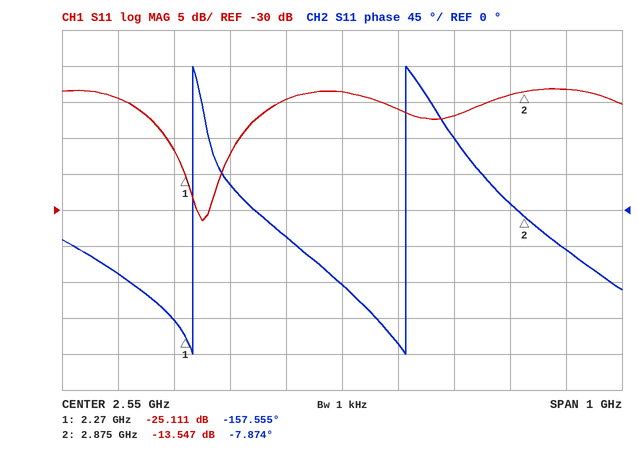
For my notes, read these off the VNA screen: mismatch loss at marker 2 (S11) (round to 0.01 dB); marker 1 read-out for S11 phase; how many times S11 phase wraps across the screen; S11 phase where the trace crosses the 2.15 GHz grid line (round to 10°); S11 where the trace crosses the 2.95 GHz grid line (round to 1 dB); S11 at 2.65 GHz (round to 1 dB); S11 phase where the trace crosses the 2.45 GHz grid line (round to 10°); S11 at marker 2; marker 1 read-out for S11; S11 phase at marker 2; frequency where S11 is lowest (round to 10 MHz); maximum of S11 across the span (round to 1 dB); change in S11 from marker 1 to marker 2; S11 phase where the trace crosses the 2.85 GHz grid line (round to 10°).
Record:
0.20 dB
-157.555°
2
-80°
-13 dB
-16 dB
-30°
-13.547 dB
-25.111 dB
-7.874°
2.30 GHz
-13 dB
11.564 dB
10°
